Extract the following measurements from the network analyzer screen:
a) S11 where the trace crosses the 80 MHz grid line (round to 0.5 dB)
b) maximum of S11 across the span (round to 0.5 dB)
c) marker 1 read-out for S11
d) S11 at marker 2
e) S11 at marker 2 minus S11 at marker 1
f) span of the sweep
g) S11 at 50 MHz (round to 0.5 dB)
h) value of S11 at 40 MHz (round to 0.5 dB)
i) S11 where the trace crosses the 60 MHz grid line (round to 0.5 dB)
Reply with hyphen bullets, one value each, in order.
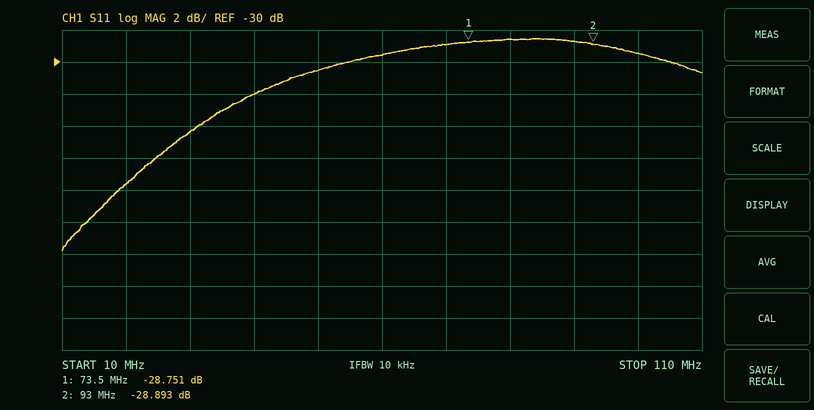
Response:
- -28.5 dB
- -28.5 dB
- -28.751 dB
- -28.893 dB
- -0.142 dB
- 100 MHz
- -30.5 dB
- -32.0 dB
- -29.5 dB
